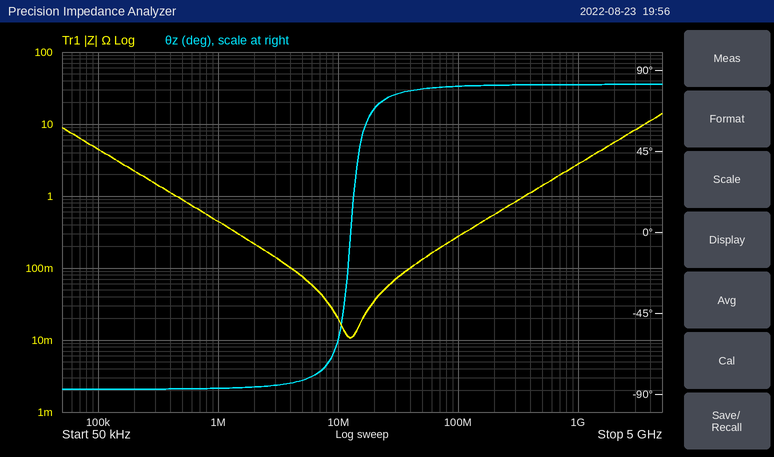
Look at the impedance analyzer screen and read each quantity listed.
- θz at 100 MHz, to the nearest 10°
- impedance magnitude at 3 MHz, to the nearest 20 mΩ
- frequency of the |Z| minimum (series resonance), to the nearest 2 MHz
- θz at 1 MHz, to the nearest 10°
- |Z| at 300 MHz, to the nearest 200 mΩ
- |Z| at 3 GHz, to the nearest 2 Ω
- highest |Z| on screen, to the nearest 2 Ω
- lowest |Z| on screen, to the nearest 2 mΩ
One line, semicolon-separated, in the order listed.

80°; 140 mΩ; 12 MHz; -90°; 800 mΩ; 8 Ω; 14 Ω; 10 mΩ
